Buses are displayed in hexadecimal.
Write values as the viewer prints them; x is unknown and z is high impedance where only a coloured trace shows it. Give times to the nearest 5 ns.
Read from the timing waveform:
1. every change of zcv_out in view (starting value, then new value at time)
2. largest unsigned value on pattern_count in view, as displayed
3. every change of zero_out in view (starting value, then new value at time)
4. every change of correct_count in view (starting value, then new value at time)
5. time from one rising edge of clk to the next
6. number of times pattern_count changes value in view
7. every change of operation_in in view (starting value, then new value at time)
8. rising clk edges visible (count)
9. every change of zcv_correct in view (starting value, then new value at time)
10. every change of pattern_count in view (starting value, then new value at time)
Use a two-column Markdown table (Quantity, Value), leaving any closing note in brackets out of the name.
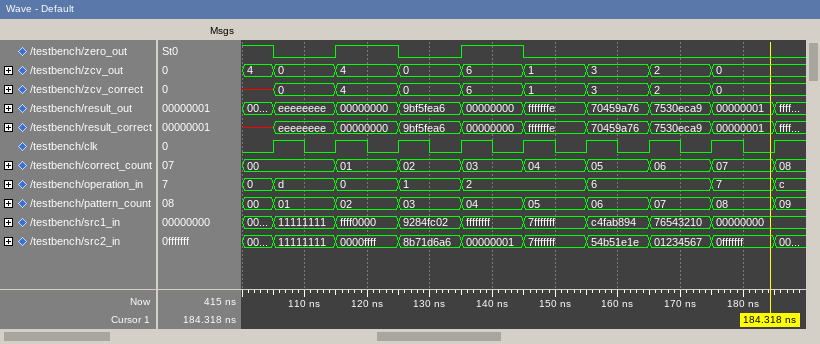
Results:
| Quantity | Value |
|---|---|
| every change of zcv_out in view | 4, 0 at 105 ns, 4 at 115 ns, 0 at 125 ns, 6 at 135 ns, 1 at 145 ns, 3 at 155 ns, 2 at 165 ns, 0 at 175 ns |
| largest unsigned value on pattern_count in view, as displayed | 09 |
| every change of zero_out in view | 1, 0 at 105 ns, 1 at 115 ns, 0 at 125 ns, 1 at 135 ns, 0 at 145 ns |
| every change of correct_count in view | 00, 01 at 115 ns, 02 at 125 ns, 03 at 135 ns, 04 at 145 ns, 05 at 155 ns, 06 at 165 ns, 07 at 175 ns, 08 at 185 ns |
| time from one rising edge of clk to the next | 10 ns |
| number of times pattern_count changes value in view | 9 |
| every change of operation_in in view | 0, d at 105 ns, 0 at 115 ns, 1 at 125 ns, 2 at 135 ns, 6 at 155 ns, 7 at 175 ns, c at 185 ns |
| rising clk edges visible | 9 |
| every change of zcv_correct in view | x, 0 at 105 ns, 4 at 115 ns, 0 at 125 ns, 6 at 135 ns, 1 at 145 ns, 3 at 155 ns, 2 at 165 ns, 0 at 175 ns |
| every change of pattern_count in view | 00, 01 at 105 ns, 02 at 115 ns, 03 at 125 ns, 04 at 135 ns, 05 at 145 ns, 06 at 155 ns, 07 at 165 ns, 08 at 175 ns, 09 at 185 ns |
